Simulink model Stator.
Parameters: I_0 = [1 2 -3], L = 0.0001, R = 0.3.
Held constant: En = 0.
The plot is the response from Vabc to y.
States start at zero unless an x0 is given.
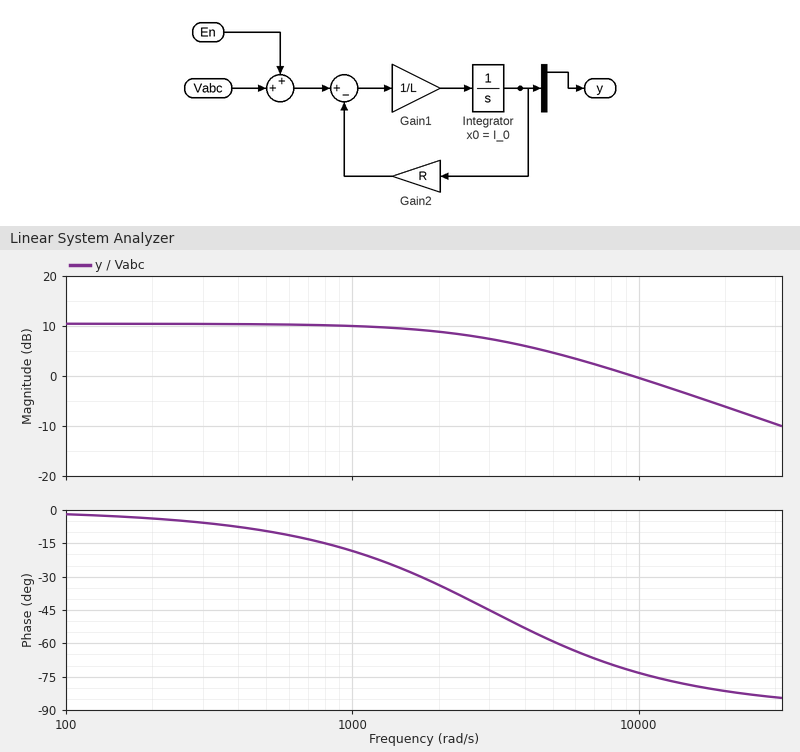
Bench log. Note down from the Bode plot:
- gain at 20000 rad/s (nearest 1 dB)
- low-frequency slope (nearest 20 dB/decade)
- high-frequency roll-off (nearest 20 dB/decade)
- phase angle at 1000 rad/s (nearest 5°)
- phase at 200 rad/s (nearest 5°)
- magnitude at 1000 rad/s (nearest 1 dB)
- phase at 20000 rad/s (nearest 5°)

-6 dB
0 dB/decade
-20 dB/decade
-20°
-5°
10 dB
-80°
